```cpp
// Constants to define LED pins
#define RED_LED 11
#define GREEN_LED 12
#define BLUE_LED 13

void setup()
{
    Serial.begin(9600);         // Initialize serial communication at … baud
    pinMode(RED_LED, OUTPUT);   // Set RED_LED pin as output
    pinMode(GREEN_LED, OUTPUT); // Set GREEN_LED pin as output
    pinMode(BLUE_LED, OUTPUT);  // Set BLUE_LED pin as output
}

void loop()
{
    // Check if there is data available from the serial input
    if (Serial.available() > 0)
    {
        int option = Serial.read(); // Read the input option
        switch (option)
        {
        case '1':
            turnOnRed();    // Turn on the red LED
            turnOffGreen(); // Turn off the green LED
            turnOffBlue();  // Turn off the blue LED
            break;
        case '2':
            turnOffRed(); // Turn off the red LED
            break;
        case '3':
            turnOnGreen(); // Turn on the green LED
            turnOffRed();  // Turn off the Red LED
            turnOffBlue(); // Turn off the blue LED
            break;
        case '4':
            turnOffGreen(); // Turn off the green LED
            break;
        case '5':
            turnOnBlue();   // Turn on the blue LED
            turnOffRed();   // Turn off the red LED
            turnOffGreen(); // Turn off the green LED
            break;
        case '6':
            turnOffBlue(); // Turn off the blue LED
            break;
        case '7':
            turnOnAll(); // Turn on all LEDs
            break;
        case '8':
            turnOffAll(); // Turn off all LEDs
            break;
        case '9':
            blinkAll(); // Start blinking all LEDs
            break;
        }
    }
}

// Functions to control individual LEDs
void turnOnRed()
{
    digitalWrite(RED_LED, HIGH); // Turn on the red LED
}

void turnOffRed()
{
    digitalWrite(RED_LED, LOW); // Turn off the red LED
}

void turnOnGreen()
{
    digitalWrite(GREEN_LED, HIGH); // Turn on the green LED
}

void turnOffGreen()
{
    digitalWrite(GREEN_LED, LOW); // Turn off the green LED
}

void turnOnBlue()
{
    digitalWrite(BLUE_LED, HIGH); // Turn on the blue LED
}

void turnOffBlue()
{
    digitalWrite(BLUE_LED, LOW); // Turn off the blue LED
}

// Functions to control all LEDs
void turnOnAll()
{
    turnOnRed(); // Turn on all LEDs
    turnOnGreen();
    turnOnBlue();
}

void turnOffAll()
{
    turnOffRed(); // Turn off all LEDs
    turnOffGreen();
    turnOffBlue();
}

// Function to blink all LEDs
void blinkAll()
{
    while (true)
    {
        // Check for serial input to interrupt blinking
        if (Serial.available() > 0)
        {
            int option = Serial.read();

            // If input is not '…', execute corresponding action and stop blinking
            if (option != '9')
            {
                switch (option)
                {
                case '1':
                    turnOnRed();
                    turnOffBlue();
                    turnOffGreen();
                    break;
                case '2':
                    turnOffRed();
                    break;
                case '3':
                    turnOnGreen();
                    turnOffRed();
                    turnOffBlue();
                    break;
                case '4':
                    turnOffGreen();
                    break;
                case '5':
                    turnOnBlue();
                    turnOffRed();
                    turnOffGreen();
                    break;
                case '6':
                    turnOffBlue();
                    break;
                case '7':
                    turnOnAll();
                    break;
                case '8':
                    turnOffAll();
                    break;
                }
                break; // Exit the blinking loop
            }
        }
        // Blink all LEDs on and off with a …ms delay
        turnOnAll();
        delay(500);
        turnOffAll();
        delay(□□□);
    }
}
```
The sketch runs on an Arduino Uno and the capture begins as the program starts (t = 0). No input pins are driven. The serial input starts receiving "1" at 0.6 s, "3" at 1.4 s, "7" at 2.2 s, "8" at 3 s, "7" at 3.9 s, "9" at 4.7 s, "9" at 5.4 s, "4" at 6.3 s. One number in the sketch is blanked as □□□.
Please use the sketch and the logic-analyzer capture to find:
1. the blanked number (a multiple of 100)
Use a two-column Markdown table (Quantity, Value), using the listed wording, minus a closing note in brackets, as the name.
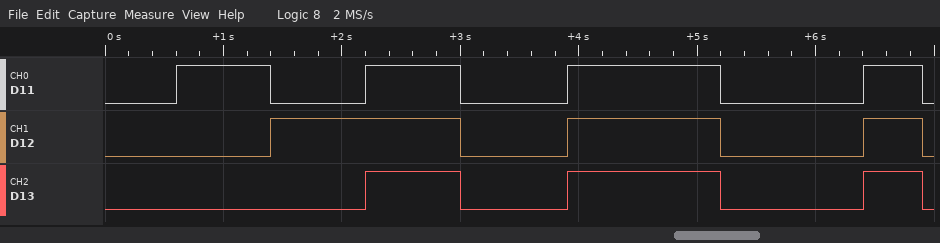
| Quantity | Value |
|---|---|
| the blanked number | 1200 |
